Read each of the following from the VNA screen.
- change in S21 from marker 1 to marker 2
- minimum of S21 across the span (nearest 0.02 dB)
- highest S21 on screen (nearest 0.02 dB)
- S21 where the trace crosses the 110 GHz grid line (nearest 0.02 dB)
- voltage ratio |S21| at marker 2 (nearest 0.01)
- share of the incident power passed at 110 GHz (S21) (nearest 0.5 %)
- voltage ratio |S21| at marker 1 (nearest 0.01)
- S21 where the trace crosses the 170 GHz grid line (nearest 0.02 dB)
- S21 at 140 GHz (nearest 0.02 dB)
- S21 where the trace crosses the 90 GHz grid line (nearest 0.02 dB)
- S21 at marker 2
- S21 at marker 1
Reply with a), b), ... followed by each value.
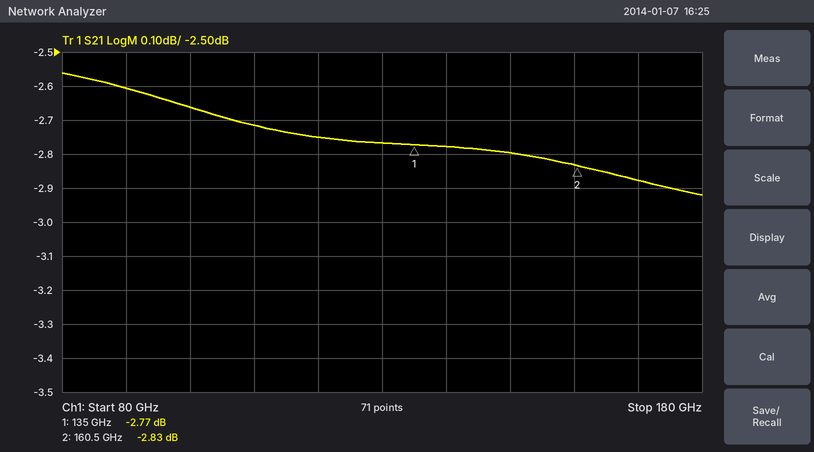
a) -0.06 dB
b) -2.92 dB
c) -2.56 dB
d) -2.72 dB
e) 0.72
f) 53.5 %
g) 0.73
h) -2.88 dB
i) -2.78 dB
j) -2.60 dB
k) -2.83 dB
l) -2.77 dB
